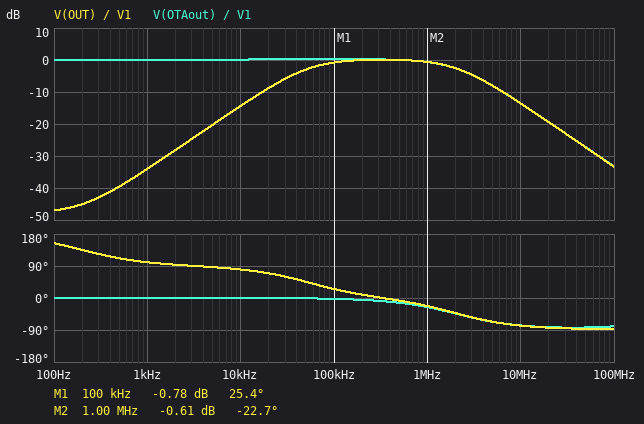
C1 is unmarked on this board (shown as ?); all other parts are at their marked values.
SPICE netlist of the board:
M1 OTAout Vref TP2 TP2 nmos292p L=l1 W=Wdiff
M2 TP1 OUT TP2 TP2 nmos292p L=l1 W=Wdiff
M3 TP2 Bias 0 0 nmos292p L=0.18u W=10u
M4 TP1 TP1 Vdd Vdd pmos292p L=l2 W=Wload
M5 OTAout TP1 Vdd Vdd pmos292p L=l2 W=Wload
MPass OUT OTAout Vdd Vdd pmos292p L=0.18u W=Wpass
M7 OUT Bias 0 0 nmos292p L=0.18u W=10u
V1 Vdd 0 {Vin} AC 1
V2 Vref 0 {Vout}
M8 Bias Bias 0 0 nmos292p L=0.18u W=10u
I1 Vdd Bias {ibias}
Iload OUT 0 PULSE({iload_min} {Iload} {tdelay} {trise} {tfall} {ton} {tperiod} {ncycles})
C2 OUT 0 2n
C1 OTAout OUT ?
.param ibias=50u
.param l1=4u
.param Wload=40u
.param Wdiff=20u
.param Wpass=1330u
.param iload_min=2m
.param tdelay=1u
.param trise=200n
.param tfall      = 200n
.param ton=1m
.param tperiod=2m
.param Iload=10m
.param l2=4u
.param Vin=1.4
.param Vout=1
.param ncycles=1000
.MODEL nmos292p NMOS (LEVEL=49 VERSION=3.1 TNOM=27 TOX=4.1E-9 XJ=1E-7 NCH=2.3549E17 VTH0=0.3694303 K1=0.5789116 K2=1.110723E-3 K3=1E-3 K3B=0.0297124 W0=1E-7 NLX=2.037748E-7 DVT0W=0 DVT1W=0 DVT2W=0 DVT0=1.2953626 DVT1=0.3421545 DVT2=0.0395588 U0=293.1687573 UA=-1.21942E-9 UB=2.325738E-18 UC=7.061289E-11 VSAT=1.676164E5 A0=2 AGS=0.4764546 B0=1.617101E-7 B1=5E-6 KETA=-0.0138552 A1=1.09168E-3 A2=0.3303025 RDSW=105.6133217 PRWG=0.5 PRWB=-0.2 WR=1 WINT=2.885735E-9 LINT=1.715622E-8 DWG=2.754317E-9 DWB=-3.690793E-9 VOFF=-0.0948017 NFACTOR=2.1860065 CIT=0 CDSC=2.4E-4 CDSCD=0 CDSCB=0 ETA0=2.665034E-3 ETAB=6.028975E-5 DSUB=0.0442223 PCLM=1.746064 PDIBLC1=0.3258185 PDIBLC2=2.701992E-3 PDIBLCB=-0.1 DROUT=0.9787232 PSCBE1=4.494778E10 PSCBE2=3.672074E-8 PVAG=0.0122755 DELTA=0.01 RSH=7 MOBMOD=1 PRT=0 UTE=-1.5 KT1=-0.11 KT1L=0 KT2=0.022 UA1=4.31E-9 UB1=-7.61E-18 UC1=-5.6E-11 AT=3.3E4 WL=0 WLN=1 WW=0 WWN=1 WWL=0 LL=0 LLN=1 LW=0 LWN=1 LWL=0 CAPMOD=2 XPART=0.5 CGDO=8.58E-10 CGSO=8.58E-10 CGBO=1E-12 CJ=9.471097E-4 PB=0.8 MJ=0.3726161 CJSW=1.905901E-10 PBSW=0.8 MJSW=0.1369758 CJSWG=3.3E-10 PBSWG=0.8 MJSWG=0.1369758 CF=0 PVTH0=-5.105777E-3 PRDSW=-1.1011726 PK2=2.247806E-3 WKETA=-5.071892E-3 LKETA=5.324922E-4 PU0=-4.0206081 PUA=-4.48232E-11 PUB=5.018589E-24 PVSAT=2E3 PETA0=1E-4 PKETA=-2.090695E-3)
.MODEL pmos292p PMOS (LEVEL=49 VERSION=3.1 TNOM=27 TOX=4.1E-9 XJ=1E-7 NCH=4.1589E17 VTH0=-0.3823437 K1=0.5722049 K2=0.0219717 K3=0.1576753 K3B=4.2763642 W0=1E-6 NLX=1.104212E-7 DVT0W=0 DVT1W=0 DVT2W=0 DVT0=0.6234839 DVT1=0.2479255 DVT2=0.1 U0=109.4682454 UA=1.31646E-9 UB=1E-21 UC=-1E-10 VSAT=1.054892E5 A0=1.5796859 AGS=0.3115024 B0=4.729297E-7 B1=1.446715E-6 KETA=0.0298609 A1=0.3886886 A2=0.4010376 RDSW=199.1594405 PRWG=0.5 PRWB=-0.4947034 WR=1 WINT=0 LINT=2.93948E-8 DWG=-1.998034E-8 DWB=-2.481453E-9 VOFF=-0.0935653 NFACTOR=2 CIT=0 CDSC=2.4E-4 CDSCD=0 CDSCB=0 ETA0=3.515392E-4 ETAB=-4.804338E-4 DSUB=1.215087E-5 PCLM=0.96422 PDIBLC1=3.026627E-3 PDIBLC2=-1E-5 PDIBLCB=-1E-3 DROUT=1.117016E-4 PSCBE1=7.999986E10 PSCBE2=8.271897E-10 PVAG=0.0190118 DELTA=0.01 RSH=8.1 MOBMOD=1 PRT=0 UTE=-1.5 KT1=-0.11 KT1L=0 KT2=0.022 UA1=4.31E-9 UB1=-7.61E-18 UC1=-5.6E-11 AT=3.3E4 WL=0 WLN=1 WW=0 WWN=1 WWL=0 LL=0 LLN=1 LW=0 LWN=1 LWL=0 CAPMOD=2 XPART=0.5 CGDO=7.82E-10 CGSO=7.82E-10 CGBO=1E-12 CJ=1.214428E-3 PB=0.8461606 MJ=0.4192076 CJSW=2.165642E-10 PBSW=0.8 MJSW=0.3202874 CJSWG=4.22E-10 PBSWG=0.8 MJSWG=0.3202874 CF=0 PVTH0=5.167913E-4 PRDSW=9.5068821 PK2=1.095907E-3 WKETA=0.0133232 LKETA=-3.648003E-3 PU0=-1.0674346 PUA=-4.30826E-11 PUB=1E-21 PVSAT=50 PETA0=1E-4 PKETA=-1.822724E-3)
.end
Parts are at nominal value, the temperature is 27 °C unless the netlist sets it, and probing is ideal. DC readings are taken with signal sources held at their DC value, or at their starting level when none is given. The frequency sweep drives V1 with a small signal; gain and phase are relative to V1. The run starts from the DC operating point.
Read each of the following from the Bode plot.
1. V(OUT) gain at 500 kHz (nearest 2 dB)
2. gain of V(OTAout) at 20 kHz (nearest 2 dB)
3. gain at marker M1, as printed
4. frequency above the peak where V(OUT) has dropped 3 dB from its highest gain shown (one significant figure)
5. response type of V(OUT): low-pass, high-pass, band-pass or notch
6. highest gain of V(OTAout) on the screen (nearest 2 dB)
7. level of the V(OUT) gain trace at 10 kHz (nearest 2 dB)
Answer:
0 dB
0 dB
-0.78 dB
2 MHz
band-pass
0 dB
-14 dB
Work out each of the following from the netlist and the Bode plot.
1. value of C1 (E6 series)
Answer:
680 pF
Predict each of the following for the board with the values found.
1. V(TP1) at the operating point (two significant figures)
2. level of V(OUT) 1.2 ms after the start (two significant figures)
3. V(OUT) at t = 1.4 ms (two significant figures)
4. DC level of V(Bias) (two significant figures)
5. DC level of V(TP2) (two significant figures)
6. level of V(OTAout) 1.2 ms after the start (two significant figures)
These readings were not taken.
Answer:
720 mV
1.0 V
1.0 V
540 mV
410 mV
840 mV
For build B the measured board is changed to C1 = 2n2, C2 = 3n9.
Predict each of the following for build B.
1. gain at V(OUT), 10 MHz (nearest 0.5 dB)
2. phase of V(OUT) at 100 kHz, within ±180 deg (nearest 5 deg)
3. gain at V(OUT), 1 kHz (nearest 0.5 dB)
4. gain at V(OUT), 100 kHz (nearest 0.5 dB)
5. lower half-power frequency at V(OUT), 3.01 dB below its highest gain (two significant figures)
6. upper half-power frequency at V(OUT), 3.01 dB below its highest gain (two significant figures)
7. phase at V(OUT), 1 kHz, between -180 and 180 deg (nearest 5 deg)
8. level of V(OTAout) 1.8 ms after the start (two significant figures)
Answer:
-19.0 dB
5 deg
-24.0 dB
0 dB
16 kHz
1.1 MHz
90 deg
840 mV
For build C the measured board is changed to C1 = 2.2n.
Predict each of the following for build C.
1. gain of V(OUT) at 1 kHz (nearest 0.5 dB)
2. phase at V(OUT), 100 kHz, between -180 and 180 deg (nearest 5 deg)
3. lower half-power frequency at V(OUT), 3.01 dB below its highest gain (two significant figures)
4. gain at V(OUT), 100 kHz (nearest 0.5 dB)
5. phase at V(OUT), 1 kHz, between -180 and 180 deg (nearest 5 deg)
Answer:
-24.0 dB
5 deg
16 kHz
0 dB
90 deg
